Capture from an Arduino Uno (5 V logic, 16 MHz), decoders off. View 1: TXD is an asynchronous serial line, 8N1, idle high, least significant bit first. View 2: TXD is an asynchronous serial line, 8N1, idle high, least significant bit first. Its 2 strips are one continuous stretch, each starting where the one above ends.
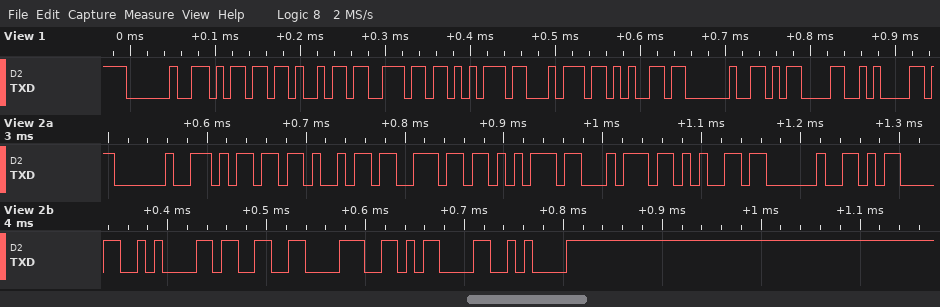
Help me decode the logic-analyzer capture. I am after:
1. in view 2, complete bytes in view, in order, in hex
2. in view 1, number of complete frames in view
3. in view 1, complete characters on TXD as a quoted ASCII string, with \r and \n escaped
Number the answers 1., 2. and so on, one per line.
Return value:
1. 0x20 0x6D 0x69 0x6E 0x75 0x74 0x65 0x20 0x0D 0x0A 0x33 0x38 0x0D 0x0A
2. 10
3. " minute \r\n"
